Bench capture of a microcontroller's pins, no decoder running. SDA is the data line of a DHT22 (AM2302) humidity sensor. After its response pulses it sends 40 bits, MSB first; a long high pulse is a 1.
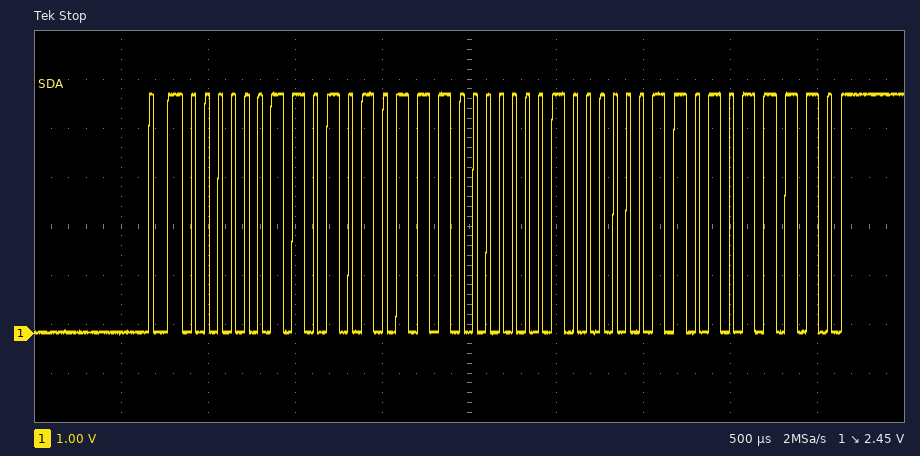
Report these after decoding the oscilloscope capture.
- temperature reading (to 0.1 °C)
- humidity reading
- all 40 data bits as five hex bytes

25.9 °C
85.5 %
03 57 01 03 5E
